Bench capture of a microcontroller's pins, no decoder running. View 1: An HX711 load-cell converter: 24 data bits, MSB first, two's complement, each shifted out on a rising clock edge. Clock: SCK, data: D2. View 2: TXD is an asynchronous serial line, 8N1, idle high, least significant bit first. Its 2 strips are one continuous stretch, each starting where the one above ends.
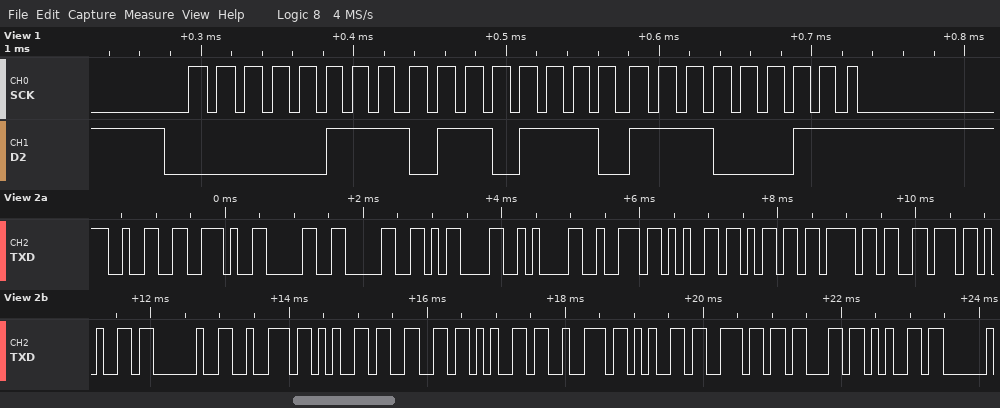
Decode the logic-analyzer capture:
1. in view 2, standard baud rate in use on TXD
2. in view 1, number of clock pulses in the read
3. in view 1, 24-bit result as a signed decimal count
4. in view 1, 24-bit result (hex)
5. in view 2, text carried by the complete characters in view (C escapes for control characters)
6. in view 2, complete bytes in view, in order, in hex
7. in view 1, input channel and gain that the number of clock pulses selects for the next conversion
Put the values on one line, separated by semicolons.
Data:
9600 baud; 25; 487139; 0x076EE3; "2.00\r\nremove reference"; 32 2E 30 30 0D 0A 72 65 6D 6F 76 65 20 72 65 66 65 72 65 6E 63 65; channel A, gain 128
